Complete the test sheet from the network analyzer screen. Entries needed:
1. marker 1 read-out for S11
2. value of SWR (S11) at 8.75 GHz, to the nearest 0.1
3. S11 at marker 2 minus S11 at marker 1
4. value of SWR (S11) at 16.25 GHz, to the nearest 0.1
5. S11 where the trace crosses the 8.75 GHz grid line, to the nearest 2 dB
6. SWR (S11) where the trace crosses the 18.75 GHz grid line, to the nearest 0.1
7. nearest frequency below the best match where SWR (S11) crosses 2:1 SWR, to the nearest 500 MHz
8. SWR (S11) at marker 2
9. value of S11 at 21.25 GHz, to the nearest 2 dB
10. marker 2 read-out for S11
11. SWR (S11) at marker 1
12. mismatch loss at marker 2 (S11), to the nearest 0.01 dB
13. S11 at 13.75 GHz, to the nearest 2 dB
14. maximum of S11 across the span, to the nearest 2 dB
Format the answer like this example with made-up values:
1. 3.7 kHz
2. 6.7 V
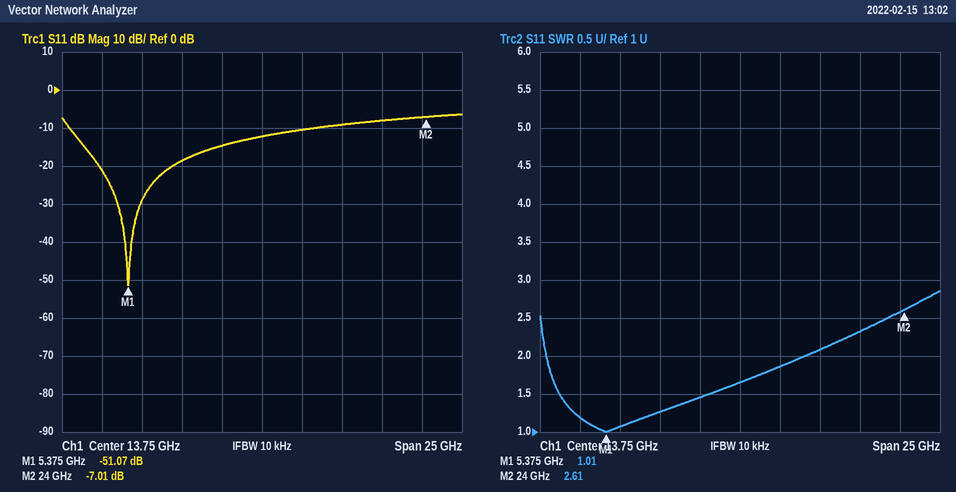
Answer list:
1. -51.07 dB
2. 1.3
3. 44.06 dB
4. 1.9
5. -18 dB
6. 2.1
7. 1.5 GHz
8. 2.61
9. -8 dB
10. -7.01 dB
11. 1.01
12. 0.96 dB
13. -12 dB
14. -6 dB
